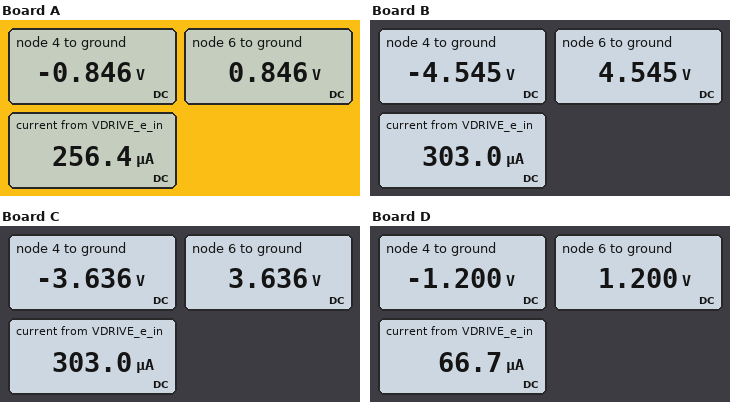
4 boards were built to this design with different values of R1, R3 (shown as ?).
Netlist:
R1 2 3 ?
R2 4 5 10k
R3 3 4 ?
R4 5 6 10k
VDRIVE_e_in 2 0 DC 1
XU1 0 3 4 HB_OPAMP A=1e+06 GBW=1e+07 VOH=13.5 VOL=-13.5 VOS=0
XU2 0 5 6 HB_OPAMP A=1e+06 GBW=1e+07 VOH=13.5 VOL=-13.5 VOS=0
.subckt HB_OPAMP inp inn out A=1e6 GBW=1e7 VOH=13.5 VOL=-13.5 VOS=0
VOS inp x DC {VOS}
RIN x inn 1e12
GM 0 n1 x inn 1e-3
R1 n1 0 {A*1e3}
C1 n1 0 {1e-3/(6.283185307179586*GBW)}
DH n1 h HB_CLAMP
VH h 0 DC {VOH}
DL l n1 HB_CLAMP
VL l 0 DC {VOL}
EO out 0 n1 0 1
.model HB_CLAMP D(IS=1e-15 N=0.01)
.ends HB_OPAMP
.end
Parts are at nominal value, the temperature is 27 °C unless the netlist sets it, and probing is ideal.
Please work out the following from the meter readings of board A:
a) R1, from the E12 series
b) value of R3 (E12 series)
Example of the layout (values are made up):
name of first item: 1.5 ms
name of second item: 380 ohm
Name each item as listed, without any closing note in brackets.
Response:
R1, from the E12 series: 3.9 kΩ
value of R3: 3.3 kΩ
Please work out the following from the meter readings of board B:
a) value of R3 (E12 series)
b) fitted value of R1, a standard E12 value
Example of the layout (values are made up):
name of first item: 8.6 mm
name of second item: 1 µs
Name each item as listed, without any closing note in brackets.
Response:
value of R3: 15 kΩ
fitted value of R1, a standard E12 value: 3.3 kΩ
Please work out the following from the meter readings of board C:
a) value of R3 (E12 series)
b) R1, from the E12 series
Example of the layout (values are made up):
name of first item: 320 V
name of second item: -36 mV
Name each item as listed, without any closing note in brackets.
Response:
value of R3: 12 kΩ
R1, from the E12 series: 3.3 kΩ
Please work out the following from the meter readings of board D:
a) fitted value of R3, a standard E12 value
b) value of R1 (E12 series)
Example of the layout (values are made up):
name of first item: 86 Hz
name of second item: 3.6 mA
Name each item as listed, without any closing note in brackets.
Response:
fitted value of R3, a standard E12 value: 18 kΩ
value of R1: 15 kΩ
